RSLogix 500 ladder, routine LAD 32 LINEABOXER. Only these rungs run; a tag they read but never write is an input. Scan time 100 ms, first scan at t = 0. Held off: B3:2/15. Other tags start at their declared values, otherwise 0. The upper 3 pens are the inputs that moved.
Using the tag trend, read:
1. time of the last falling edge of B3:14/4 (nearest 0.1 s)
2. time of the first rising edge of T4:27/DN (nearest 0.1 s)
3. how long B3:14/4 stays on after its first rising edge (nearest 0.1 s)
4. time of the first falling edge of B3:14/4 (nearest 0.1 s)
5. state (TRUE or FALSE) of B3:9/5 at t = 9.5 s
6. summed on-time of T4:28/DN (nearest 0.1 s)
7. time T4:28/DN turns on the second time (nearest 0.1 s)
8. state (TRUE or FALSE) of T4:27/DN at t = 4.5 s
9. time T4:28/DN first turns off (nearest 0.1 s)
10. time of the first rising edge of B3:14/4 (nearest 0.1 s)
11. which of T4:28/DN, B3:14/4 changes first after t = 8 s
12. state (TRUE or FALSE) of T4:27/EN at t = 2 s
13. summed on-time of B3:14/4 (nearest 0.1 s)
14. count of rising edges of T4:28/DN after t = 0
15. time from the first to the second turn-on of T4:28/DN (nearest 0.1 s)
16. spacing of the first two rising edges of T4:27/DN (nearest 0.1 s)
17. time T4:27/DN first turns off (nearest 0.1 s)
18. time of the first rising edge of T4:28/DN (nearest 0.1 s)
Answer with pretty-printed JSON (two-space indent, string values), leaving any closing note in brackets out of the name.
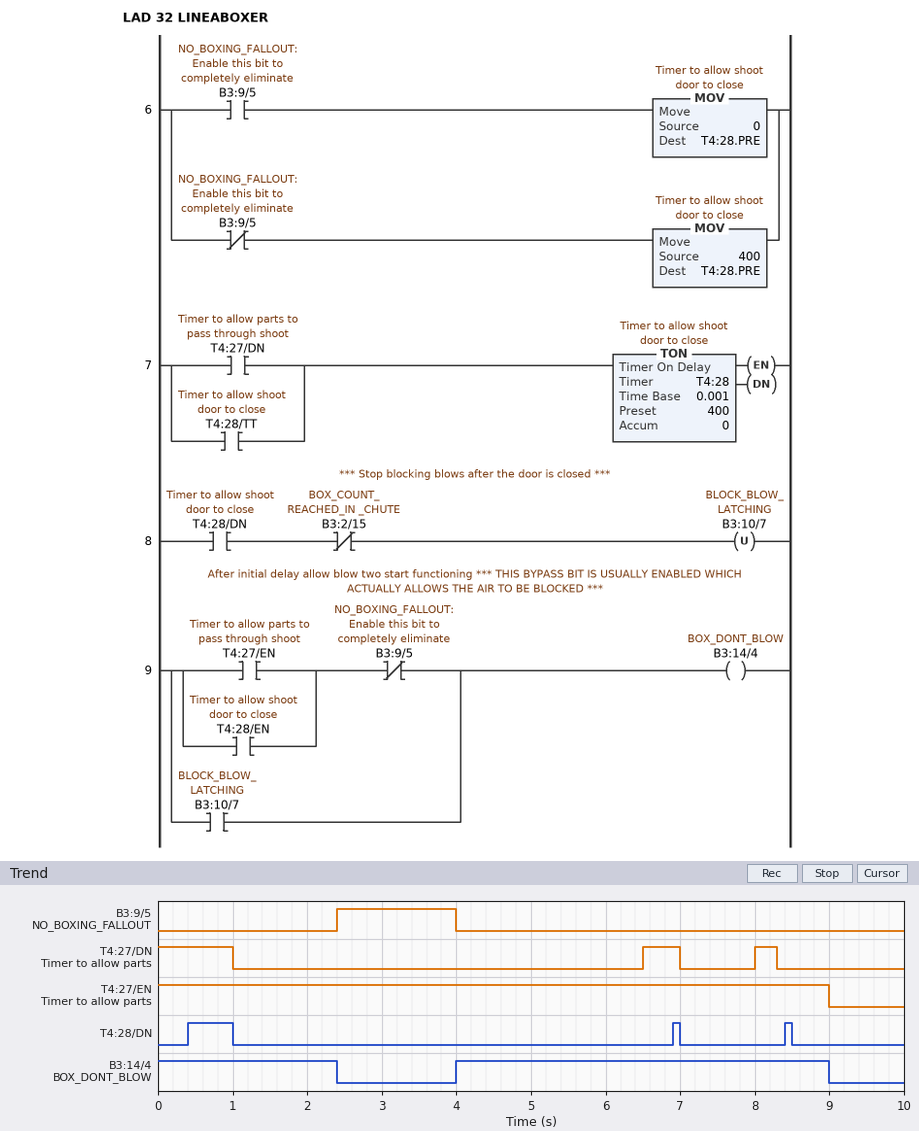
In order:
{
  "time of the last falling edge of B3:14/4": "9.0 s",
  "time of the first rising edge of T4:27/DN": "6.5 s",
  "how long B3:14/4 stays on after its first rising edge": "5.0 s",
  "time of the first falling edge of B3:14/4": "2.4 s",
  "state (TRUE or FALSE) of B3:9/5 at t = 9.5 s": "FALSE",
  "summed on-time of T4:28/DN": "0.8 s",
  "time T4:28/DN turns on the second time": "6.9 s",
  "state (TRUE or FALSE) of T4:27/DN at t = 4.5 s": "FALSE",
  "time T4:28/DN first turns off": "1.0 s",
  "time of the first rising edge of B3:14/4": "4.0 s",
  "which of T4:28/DN, B3:14/4 changes first after t = 8 s": "T4:28/DN",
  "state (TRUE or FALSE) of T4:27/EN at t = 2 s": "TRUE",
  "summed on-time of B3:14/4": "7.4 s",
  "count of rising edges of T4:28/DN after t = 0": "3",
  "time from the first to the second turn-on of T4:28/DN": "6.5 s",
  "spacing of the first two rising edges of T4:27/DN": "1.5 s",
  "time T4:27/DN first turns off": "1.0 s",
  "time of the first rising edge of T4:28/DN": "0.4 s"
}
